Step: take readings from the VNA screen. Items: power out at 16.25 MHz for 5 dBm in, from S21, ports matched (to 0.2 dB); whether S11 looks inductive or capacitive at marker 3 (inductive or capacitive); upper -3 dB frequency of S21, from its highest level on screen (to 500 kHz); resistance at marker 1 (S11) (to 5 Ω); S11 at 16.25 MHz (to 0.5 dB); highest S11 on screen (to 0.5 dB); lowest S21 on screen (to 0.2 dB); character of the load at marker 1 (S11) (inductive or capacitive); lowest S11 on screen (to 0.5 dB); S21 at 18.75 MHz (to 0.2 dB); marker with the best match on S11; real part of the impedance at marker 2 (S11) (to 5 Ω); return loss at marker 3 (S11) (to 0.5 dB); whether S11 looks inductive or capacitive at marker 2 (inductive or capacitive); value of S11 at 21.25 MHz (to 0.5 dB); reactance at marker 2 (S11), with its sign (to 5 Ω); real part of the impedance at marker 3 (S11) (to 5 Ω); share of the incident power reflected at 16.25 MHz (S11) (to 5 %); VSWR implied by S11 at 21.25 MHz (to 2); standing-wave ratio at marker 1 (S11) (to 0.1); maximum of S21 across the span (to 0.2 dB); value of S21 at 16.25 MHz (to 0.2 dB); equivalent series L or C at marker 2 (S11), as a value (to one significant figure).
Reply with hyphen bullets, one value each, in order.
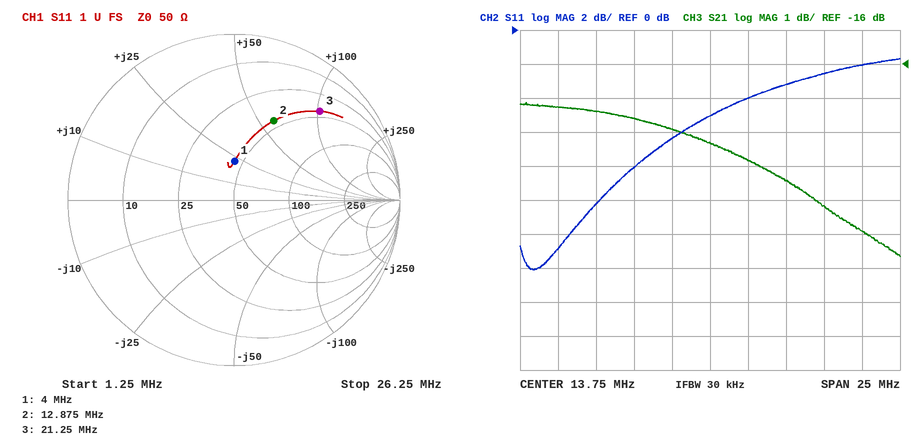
- -13.8 dBm
- inductive
- 21.0 MHz
- 45 Ω
- -4.0 dB
- -1.5 dB
- -21.6 dB
- inductive
- -14.0 dB
- -19.4 dB
- marker 1
- 45 Ω
- 2.5 dB
- inductive
- -2.5 dB
- +60 Ω
- 45 Ω
- 40 %
- 6
- 1.6
- -17.2 dB
- -18.8 dB
- 700 nH
